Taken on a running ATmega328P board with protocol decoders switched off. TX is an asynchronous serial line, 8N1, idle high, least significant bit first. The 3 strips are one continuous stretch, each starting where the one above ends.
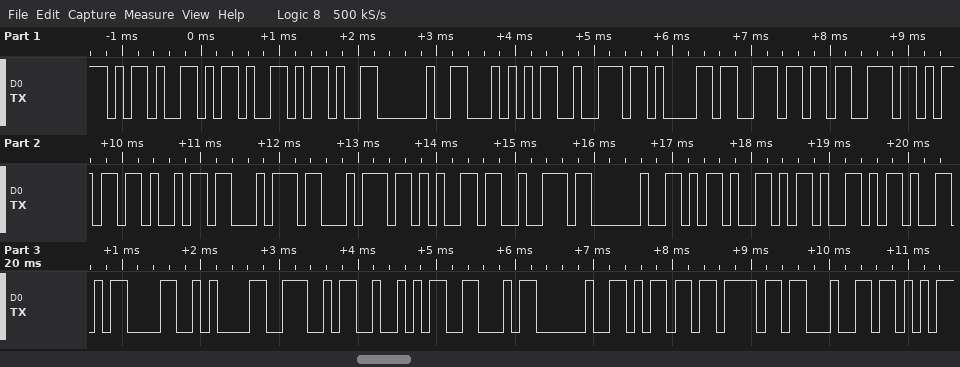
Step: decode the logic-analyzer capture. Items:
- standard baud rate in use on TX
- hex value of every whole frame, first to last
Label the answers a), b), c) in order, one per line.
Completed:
a) 9600 baud
b) 0x2D 0x2D 0x2D 0x20 0x54 0x72 0x61 0x6E 0x73 0x6D 0x69 0x74 0x74 0x65 0x72 0x20 0x2D 0x2D 0x2D 0x0D 0x0A 0x4E 0x52 0x46 0x20 0x6D 0x6F 0x64
